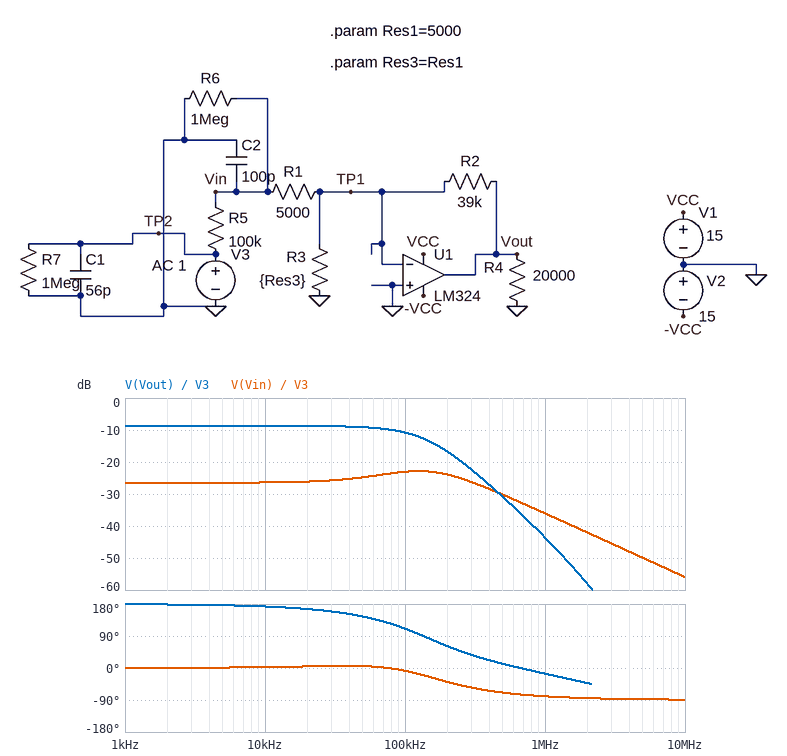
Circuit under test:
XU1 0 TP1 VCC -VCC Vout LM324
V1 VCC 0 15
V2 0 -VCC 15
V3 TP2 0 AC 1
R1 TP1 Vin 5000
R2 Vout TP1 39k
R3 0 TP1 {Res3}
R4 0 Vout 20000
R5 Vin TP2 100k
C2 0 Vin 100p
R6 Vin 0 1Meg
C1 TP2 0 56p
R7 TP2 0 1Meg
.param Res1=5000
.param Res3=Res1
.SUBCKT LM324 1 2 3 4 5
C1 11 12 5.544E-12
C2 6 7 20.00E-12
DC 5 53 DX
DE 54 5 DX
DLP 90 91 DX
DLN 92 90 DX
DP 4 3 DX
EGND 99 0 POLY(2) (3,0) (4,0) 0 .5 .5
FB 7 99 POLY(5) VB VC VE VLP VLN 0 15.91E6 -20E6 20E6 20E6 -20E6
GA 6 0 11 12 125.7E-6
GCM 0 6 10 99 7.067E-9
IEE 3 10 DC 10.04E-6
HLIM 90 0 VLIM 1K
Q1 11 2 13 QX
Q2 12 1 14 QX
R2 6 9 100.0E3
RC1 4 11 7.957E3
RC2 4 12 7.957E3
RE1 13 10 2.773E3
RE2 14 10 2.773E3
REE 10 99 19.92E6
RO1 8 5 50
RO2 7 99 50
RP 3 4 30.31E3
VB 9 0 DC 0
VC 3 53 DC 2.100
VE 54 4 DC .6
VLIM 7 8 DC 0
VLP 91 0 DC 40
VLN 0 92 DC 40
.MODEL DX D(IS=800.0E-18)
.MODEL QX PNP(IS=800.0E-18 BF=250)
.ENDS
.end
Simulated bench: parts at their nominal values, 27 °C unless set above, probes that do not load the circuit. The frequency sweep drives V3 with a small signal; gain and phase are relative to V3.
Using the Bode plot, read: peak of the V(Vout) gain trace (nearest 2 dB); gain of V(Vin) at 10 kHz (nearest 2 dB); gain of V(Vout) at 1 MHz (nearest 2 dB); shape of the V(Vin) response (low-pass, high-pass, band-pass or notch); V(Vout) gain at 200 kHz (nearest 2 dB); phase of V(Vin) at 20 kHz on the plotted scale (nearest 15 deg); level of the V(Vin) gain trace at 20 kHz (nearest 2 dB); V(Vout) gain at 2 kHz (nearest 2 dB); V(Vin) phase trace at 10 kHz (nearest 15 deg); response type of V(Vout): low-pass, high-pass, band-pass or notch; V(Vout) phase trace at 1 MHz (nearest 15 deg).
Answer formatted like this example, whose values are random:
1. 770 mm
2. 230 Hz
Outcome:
1. -8 dB
2. -26 dB
3. -44 dB
4. low-pass
5. -16 dB
6. 0 deg
7. -26 dB
8. -8 dB
9. 0 deg
10. low-pass
11. -15 deg
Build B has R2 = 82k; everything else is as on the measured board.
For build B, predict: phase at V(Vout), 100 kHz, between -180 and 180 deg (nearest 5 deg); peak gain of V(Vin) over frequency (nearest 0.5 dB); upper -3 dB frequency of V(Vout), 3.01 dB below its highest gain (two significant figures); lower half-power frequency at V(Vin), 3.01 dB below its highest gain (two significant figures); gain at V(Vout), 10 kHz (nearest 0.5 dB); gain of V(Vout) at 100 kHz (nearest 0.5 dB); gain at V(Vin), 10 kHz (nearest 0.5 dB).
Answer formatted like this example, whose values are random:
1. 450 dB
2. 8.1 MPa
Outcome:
1. 85 deg
2. -22.0 dB
3. 61 kHz
4. 23 kHz
5. -2.5 dB
6. -8.5 dB
7. -26.0 dB
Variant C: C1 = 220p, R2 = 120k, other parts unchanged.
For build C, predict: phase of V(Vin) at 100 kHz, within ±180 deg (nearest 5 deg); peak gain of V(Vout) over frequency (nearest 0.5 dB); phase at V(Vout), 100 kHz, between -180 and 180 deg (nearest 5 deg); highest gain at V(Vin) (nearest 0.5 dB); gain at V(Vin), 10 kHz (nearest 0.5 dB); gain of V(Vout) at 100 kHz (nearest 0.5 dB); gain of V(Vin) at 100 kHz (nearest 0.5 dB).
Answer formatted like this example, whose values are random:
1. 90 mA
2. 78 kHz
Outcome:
1. -20 deg
2. 1.0 dB
3. 80 deg
4. -21.5 dB
5. -26.0 dB
6. -8.0 dB
7. -22.0 dB
